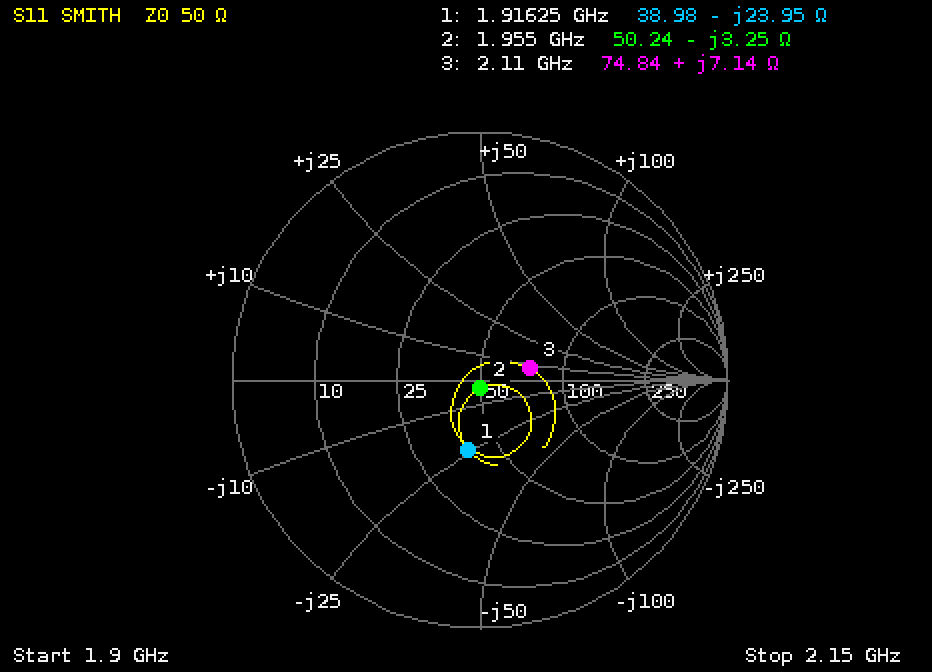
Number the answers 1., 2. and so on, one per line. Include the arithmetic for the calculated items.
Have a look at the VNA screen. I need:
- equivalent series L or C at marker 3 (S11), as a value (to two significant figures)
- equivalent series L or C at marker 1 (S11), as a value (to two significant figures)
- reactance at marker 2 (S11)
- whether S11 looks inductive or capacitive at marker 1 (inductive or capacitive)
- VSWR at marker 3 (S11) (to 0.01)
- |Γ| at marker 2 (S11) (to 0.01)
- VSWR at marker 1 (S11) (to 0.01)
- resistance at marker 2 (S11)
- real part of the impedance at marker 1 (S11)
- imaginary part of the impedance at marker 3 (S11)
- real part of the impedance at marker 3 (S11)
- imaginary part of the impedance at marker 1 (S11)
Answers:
1. L = 7.14 Ω/(2π × 2.11 GHz) ≈ 539 pH, so 540 pH to two significant figures
2. C = 1/(2π × 1.91625 GHz × 23.95 Ω) ≈ 3.5 pF
3. -3.25 Ω
4. capacitive
5. 1.52
6. 0.03
7. 1.80
8. 50.24 Ω
9. 38.98 Ω
10. +7.14 Ω
11. 74.84 Ω
12. -23.95 Ω
